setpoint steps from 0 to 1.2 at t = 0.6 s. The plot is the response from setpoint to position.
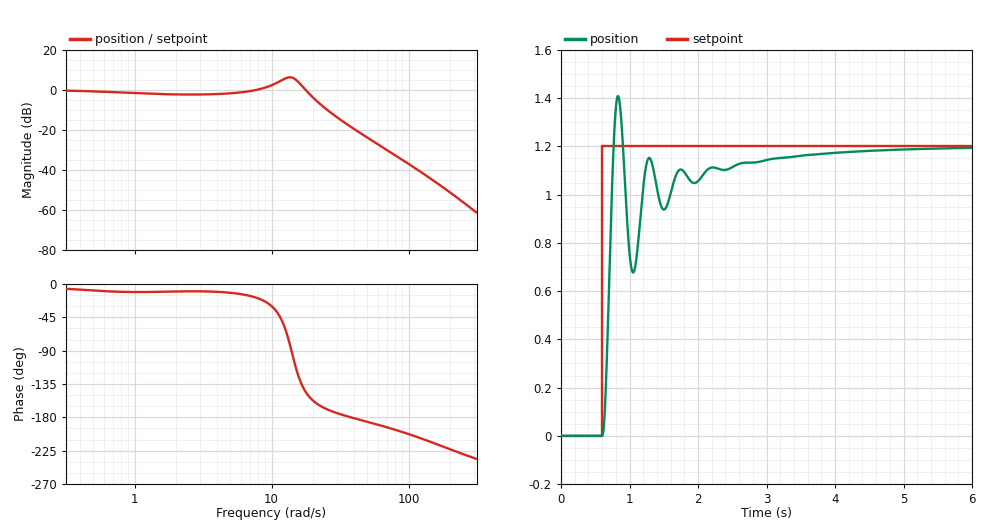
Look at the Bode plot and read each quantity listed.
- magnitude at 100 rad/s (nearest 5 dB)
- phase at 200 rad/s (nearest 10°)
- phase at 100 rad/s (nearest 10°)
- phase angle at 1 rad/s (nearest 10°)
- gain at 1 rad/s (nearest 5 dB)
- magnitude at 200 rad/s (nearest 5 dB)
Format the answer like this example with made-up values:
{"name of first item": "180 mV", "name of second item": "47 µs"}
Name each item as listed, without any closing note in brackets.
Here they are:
{"magnitude at 100 rad/s": "-35 dB", "phase at 200 rad/s": "-220°", "phase at 100 rad/s": "-200°", "phase angle at 1 rad/s": "-10°", "gain at 1 rad/s": "0 dB", "magnitude at 200 rad/s": "-50 dB"}
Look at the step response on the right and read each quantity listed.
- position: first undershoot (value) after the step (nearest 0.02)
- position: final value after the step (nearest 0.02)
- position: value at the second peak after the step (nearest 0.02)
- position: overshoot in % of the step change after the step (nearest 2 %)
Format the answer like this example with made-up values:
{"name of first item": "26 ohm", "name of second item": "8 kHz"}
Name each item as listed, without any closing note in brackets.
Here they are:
{"position: first undershoot (value) after the step": "0.68", "position: final value after the step": "1.20", "position: value at the second peak after the step": "1.16", "position: overshoot in % of the step change after the step": "18 %"}
